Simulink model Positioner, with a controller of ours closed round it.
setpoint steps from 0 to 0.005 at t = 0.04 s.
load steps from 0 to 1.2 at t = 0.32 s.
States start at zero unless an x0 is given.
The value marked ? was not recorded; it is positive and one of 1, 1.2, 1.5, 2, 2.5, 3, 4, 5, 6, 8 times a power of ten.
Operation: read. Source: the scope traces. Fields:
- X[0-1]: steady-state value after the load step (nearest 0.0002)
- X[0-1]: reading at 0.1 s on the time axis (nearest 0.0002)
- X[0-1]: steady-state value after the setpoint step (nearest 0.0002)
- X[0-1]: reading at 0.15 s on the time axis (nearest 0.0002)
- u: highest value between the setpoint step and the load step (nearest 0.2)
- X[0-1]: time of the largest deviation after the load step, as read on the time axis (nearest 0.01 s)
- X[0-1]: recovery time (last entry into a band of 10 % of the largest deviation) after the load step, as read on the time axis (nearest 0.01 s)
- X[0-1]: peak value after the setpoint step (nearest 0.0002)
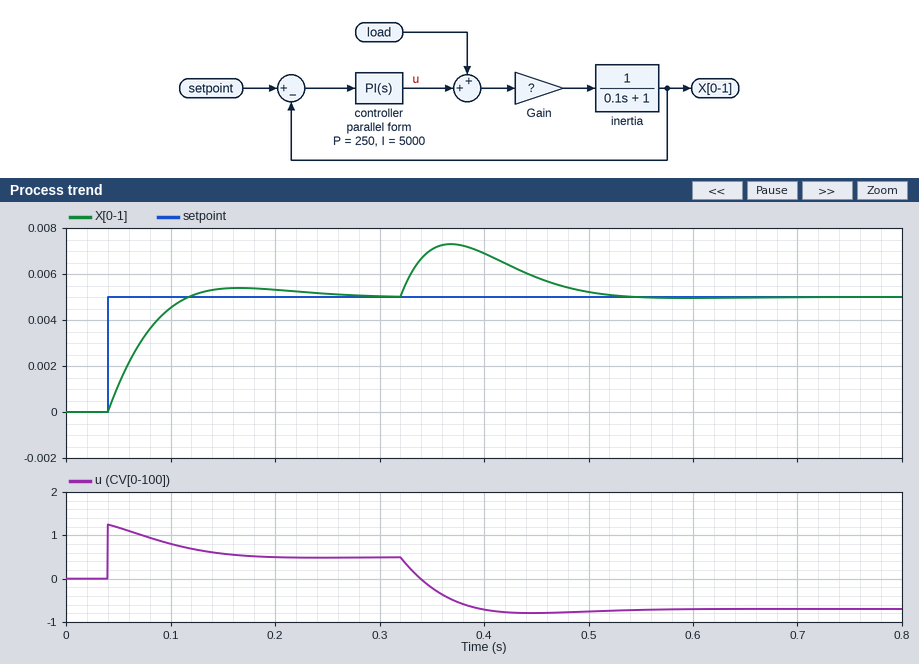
0.0050
0.0046
0.0050
0.0054
1.2
0.37 s
0.50 s
0.0054
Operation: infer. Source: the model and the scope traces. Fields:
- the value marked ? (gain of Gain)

0.01
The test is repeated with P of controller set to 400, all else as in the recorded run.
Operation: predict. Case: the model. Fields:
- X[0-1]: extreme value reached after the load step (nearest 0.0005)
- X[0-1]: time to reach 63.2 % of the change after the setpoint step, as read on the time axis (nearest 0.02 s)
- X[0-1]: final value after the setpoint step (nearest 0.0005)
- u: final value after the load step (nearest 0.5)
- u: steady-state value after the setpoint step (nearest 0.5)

0.0070
0.06 s
0.0050
-0.5
0.5
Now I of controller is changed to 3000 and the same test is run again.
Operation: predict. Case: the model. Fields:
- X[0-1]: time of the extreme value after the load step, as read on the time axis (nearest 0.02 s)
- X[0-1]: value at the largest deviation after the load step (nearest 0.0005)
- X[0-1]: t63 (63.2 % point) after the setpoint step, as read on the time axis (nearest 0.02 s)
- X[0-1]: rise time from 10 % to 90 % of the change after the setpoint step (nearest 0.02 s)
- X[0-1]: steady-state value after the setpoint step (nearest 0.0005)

0.38 s
0.0075
0.08 s
0.08 s
0.0050
